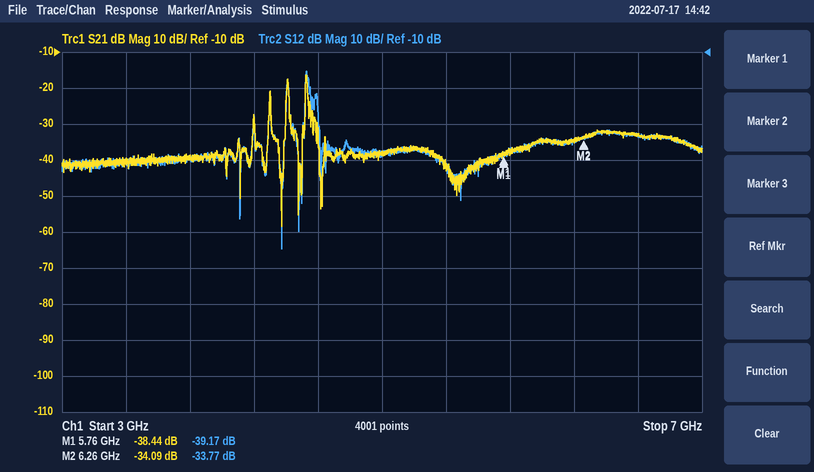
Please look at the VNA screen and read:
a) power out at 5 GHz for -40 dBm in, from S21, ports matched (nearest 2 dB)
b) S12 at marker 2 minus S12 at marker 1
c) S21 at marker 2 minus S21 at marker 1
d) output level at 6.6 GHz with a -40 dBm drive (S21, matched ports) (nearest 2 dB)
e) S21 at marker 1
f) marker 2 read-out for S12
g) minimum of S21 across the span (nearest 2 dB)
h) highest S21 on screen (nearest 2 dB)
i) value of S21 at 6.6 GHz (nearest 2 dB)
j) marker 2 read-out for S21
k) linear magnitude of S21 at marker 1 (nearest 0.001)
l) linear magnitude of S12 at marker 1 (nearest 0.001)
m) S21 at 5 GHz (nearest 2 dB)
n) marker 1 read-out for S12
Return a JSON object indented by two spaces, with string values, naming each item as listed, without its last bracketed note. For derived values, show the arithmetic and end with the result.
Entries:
{
  "power out at 5 GHz for -40 dBm in, from S21, ports matched": "-40 dBm + (-38 dB) = -78 dBm",
  "S12 at marker 2 minus S12 at marker 1": "-33.77 − (-39.17) = 5.40 dB",
  "S21 at marker 2 minus S21 at marker 1": "-34.09 − (-38.44) = 4.35 dB",
  "output level at 6.6 GHz with a -40 dBm drive (S21, matched ports)": "-40 dBm + (-32 dB) = -72 dBm",
  "S21 at marker 1": "-38.44 dB",
  "marker 2 read-out for S12": "-33.77 dB",
  "minimum of S21 across the span": "-58 dB",
  "highest S21 on screen": "-16 dB",
  "value of S21 at 6.6 GHz": "-32 dB",
  "marker 2 read-out for S21": "-34.09 dB",
  "linear magnitude of S21 at marker 1": "10^(-38.44/20) ≈ 0.012",
  "linear magnitude of S12 at marker 1": "10^(-39.17/20) ≈ 0.011",
  "S21 at 5 GHz": "-38 dB",
  "marker 1 read-out for S12": "-39.17 dB"
}
